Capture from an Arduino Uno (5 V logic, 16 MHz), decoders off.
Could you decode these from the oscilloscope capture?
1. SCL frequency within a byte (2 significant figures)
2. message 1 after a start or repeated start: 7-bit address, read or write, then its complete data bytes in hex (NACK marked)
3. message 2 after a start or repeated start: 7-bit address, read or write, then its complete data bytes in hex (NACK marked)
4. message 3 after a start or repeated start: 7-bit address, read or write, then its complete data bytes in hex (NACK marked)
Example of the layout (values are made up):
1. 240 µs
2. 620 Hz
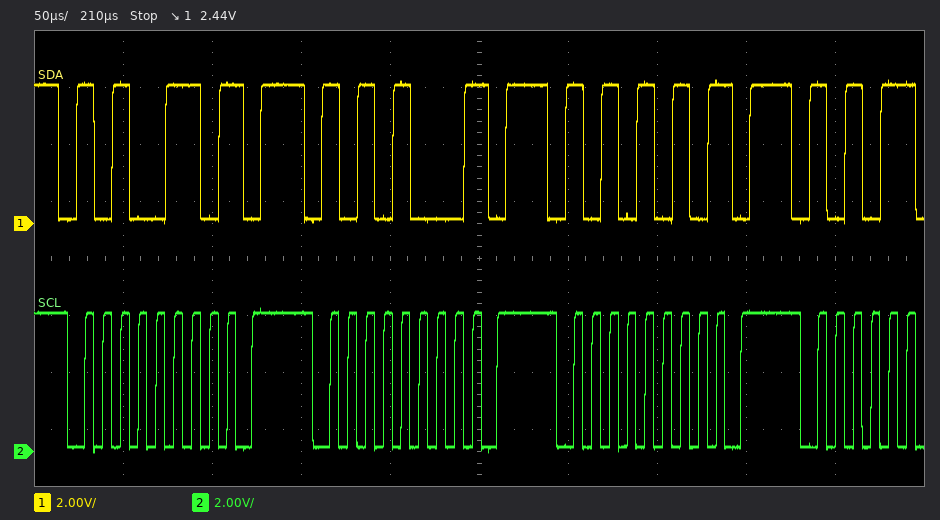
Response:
1. 100 kHz
2. 0x53 write NACK
3. 0x54 write NACK
4. 0x55 write NACK
